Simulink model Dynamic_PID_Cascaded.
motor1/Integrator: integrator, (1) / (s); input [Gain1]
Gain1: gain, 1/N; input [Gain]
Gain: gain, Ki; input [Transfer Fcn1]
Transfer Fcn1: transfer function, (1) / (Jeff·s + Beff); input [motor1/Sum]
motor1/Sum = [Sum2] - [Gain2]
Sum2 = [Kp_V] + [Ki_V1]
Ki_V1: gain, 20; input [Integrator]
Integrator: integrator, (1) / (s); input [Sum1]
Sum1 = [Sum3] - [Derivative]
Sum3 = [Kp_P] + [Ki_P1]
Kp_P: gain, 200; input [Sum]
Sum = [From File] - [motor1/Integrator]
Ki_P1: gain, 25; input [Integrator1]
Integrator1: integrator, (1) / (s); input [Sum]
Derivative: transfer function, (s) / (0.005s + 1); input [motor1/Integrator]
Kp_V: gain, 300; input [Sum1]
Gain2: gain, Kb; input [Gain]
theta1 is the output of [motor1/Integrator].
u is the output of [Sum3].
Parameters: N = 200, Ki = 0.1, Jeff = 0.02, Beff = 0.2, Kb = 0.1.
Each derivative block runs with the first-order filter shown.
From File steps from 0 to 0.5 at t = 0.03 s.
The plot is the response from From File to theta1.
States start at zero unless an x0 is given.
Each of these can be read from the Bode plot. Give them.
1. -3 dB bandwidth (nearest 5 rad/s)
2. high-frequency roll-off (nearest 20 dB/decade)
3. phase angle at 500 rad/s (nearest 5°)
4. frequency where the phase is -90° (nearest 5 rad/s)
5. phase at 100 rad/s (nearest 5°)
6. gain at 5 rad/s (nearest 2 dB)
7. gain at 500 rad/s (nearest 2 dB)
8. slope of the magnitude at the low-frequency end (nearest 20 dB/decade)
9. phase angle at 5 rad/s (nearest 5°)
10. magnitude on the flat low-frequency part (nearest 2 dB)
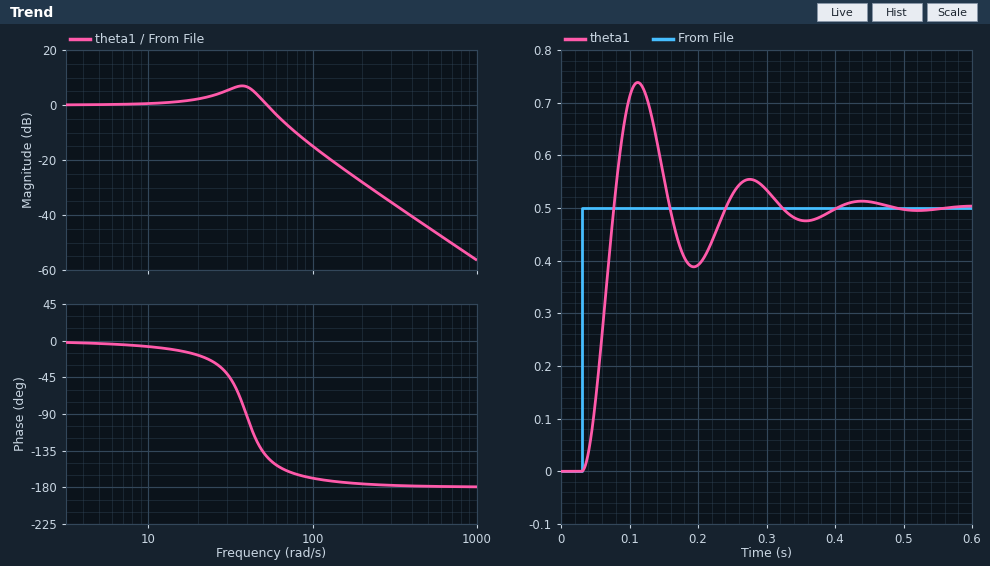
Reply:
60 rad/s
-40 dB/decade
-180°
40 rad/s
-170°
0 dB
-44 dB
0 dB/decade
-5°
0 dB
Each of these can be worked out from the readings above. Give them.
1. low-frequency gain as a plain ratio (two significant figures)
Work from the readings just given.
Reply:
1.0
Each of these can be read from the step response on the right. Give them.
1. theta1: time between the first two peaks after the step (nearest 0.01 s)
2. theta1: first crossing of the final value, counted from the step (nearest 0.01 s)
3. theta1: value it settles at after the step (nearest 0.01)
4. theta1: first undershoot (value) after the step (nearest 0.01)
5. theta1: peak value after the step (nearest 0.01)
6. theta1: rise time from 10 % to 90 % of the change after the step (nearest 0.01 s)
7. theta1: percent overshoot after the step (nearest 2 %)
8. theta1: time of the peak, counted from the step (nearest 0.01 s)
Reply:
0.16 s
0.05 s
0.50
0.39
0.74
0.03 s
48 %
0.08 s
